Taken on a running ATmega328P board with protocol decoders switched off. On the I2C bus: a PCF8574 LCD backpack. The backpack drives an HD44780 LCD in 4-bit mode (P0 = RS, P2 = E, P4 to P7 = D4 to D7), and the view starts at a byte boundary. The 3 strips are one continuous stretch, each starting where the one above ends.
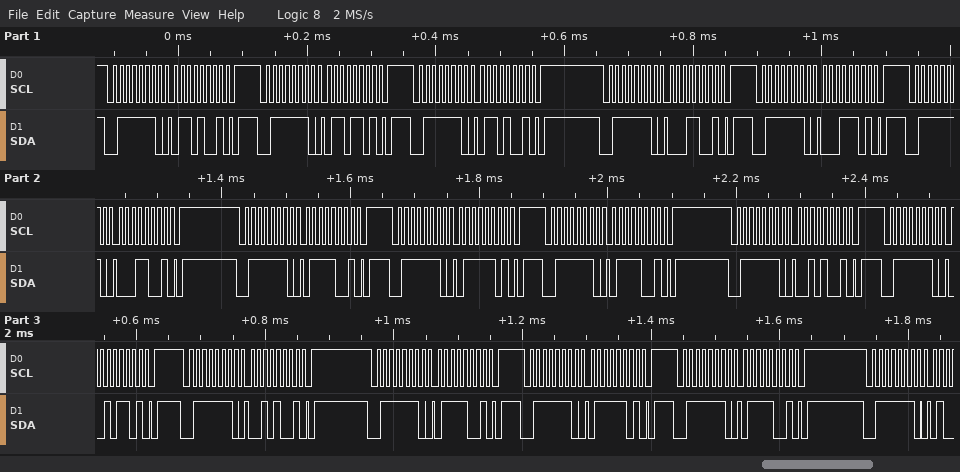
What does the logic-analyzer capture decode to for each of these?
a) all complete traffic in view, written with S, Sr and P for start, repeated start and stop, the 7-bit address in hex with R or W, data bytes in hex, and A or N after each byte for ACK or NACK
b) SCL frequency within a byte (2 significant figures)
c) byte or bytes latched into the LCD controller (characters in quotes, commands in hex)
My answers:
S 3FW A 69 A P S 3FW A 6D A P S 3FW A 69 A P S 3FW A 19 A P S 3FW A 1D A P S 3FW A 19 A P S 3FW A 79 A P S 3FW A 7D A P S 3FW A 79 A P S 3FW A 29 A P S 3FW A 2D A P S 3FW A 29 A P S 3FW A 79 A P S 3FW A 7D A P S 3FW A 79 A P S 3FW A
100 kHz
'a' 'r'
